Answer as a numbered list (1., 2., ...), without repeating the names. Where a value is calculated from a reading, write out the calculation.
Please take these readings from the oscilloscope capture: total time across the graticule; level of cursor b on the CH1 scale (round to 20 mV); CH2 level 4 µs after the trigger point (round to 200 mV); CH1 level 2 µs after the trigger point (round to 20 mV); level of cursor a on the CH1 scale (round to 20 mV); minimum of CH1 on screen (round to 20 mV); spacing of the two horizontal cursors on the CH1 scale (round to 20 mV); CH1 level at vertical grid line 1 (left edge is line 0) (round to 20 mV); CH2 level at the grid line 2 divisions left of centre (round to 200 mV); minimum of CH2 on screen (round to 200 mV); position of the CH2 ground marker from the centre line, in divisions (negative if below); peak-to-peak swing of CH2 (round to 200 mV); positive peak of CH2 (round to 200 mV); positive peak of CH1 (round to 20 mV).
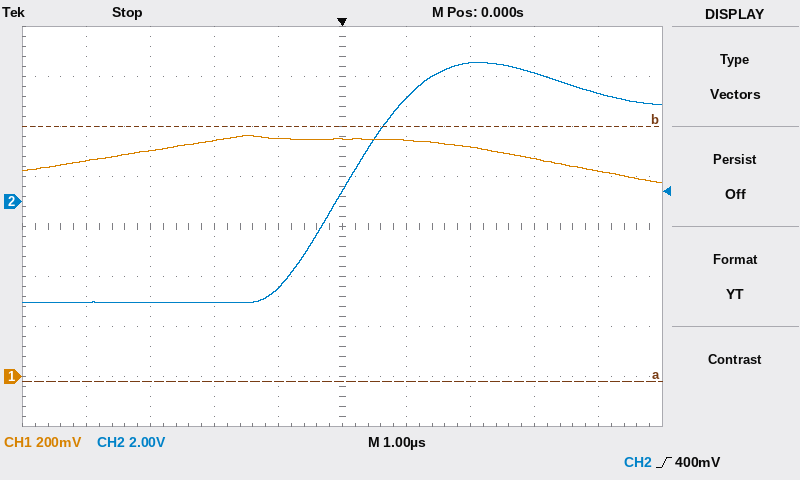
1. 10 µs
2. 1.00 V
3. 4.4 V
4. 920 mV
5. -20 mV
6. 780 mV
7. 1.02 V
8. 860 mV
9. -4.0 V
10. -4.0 V
11. +0.5 div
12. 5.6 V − (-4.0 V) = 9.6 V
13. 5.6 V
14. 960 mV
